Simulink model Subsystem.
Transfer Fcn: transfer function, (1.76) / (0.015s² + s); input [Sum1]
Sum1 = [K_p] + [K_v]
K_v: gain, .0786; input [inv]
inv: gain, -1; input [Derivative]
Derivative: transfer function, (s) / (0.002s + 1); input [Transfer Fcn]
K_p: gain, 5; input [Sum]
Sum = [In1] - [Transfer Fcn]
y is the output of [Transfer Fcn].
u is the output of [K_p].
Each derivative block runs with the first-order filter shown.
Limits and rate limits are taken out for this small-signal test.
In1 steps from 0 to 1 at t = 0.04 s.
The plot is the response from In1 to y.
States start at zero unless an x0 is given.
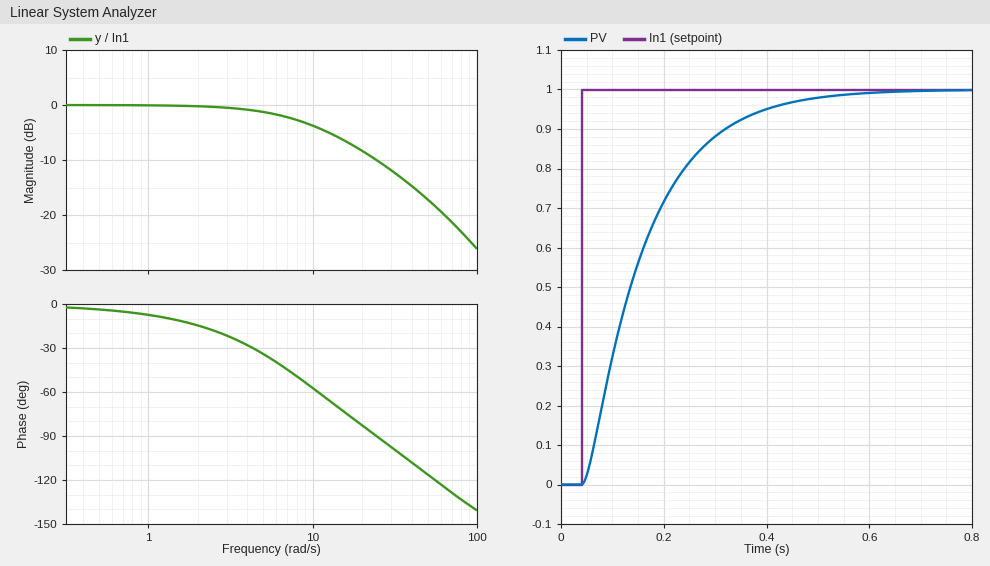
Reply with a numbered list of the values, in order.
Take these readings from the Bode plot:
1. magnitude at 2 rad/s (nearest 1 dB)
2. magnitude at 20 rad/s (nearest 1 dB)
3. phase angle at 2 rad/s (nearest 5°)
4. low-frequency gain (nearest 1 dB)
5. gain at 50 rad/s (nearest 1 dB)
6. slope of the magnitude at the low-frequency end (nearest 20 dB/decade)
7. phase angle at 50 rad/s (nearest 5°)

1. 0 dB
2. -8 dB
3. -15°
4. 0 dB
5. -17 dB
6. 0 dB/decade
7. -115°
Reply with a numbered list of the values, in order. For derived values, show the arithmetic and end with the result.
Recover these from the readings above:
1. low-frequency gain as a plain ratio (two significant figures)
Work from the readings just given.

1. 10^(0 / 20) = 1.0
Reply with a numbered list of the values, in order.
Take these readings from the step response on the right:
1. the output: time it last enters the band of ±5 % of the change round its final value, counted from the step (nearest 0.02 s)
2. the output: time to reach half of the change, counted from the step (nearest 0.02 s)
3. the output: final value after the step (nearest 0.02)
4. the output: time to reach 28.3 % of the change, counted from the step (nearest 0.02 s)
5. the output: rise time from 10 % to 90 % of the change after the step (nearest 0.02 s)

1. 0.36 s
2. 0.10 s
3. 1.00
4. 0.06 s
5. 0.26 s
